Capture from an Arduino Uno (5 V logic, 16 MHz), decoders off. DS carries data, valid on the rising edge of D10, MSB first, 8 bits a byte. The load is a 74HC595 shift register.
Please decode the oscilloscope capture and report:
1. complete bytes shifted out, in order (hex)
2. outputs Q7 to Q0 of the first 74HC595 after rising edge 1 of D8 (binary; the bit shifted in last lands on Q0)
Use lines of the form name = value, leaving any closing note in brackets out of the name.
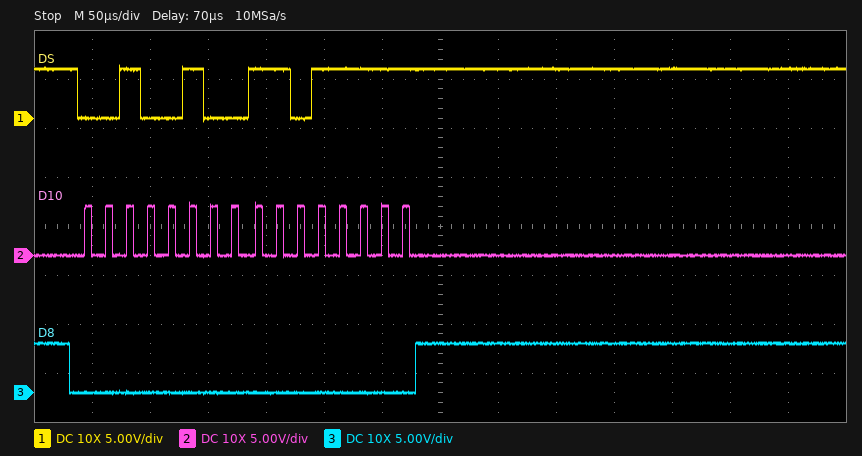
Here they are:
complete bytes shifted out, in order = 0x24 0xDF
outputs Q7 to Q0 of the first 74HC595 after rising edge 1 of D8 = 11011111
